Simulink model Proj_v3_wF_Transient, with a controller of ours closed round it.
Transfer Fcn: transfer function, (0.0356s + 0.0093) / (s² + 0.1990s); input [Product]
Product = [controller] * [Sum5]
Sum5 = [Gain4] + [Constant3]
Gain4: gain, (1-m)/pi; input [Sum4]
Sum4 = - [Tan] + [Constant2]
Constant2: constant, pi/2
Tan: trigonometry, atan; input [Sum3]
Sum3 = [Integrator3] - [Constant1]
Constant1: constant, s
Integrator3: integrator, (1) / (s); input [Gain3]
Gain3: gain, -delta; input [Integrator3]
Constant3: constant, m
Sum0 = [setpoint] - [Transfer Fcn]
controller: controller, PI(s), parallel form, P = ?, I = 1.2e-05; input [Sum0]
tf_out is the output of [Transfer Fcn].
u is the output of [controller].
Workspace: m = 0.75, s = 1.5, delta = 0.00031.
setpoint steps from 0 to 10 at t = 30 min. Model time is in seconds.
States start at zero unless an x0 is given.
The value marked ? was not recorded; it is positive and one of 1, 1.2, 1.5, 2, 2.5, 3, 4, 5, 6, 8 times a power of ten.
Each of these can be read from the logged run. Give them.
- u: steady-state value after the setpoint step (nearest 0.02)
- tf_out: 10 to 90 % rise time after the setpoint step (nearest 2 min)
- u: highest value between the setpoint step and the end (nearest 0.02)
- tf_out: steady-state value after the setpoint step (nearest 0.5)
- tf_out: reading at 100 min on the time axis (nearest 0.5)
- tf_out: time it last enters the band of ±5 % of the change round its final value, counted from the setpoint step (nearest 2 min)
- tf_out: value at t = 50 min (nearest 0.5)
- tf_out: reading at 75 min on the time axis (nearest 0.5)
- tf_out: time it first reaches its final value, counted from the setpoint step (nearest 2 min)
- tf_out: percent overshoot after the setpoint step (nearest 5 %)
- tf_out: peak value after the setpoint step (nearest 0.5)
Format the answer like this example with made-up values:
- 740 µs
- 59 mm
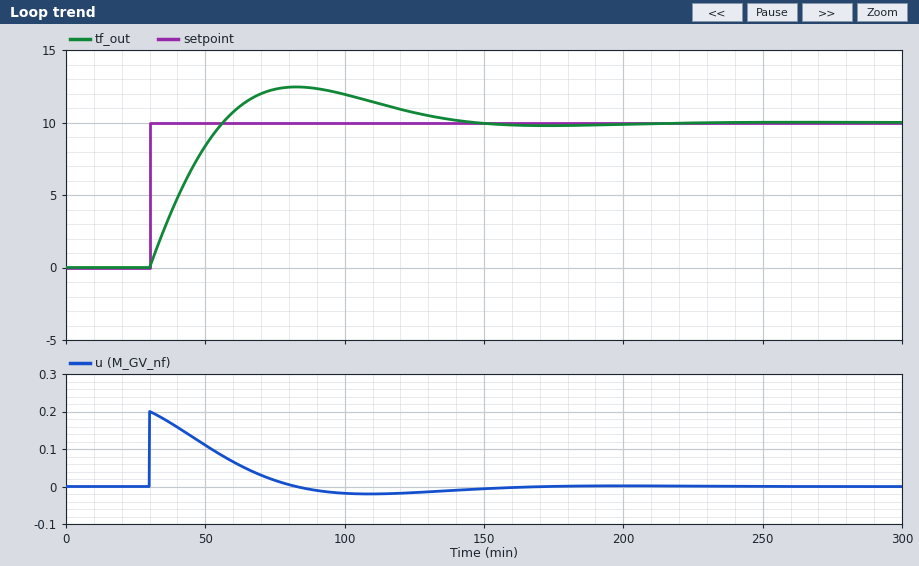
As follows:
- 0.00
- 20 min
- 0.20
- 10.0
- 12.0
- 100 min
- 8.5
- 12.5
- 26 min
- 25 %
- 12.5
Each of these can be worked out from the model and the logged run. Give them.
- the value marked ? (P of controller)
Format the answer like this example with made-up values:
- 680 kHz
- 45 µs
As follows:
- 0.02
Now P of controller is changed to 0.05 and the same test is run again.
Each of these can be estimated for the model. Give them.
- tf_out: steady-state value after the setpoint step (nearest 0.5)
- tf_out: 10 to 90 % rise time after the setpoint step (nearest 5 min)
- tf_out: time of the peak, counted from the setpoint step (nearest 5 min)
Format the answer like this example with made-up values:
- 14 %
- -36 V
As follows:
- 10.0
- 15 min
- 40 min
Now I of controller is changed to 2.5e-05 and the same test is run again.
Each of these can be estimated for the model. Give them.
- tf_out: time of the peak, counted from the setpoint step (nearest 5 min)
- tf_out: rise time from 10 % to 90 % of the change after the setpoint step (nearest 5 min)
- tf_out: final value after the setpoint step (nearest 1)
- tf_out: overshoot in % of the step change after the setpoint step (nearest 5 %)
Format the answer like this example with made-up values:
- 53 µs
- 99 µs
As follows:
- 40 min
- 15 min
- 10
- 35 %
